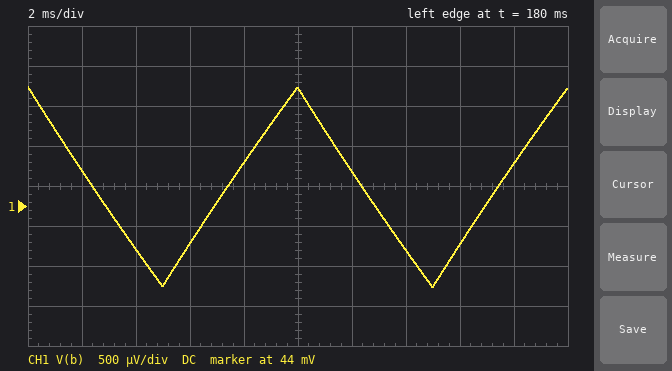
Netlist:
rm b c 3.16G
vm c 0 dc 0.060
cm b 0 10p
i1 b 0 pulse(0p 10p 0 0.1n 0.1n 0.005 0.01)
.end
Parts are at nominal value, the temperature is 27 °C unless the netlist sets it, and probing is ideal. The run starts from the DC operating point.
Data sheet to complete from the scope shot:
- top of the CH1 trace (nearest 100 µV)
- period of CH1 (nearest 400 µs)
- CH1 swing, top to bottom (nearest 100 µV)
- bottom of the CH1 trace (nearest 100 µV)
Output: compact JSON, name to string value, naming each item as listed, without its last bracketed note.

{"top of the CH1 trace": "45.5 mV", "period of CH1": "10.0 ms", "CH1 swing, top to bottom": "2.5 mV", "bottom of the CH1 trace": "43.0 mV"}
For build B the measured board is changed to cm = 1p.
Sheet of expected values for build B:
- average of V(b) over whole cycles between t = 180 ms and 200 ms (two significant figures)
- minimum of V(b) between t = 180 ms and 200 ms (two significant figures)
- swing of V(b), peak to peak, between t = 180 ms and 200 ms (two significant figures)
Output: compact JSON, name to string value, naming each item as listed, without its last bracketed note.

{"average of V(b) over whole cycles between t = 180 ms and 200 ms": "44 mV", "minimum of V(b) between t = 180 ms and 200 ms": "34 mV", "swing of V(b), peak to peak, between t = 180 ms and 200 ms": "21 mV"}
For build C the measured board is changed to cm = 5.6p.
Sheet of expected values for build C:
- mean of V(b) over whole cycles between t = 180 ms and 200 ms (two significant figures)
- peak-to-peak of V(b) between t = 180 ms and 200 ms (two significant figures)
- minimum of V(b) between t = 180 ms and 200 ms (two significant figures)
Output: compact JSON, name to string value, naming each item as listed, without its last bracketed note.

{"mean of V(b) over whole cycles between t = 180 ms and 200 ms": "44 mV", "peak-to-peak of V(b) between t = 180 ms and 200 ms": "4.4 mV", "minimum of V(b) between t = 180 ms and 200 ms": "42 mV"}
